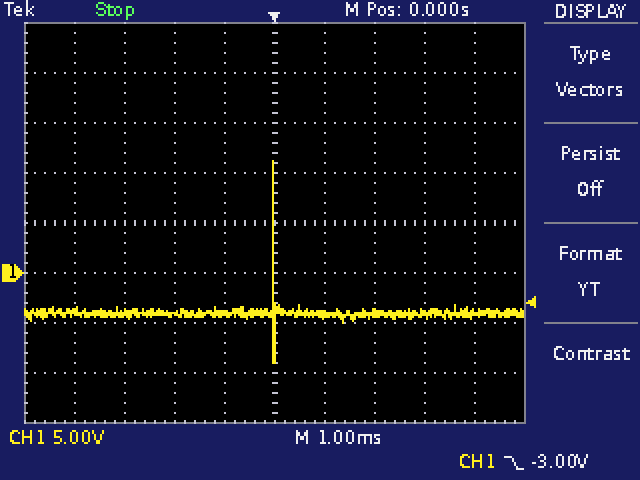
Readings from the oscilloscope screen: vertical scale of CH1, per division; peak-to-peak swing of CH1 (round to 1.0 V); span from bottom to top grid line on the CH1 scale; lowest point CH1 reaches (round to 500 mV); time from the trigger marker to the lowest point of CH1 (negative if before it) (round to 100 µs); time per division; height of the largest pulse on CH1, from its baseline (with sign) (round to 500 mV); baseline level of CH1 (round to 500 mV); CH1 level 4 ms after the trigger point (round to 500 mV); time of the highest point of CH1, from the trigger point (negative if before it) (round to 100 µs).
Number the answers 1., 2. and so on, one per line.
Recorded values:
1. 5 V
2. 20.0 V
3. 40 V
4. -9.0 V
5. 0.0 ms
6. 1 ms
7. +15.5 V
8. -4.0 V
9. -4.0 V
10. 0.0 ms
